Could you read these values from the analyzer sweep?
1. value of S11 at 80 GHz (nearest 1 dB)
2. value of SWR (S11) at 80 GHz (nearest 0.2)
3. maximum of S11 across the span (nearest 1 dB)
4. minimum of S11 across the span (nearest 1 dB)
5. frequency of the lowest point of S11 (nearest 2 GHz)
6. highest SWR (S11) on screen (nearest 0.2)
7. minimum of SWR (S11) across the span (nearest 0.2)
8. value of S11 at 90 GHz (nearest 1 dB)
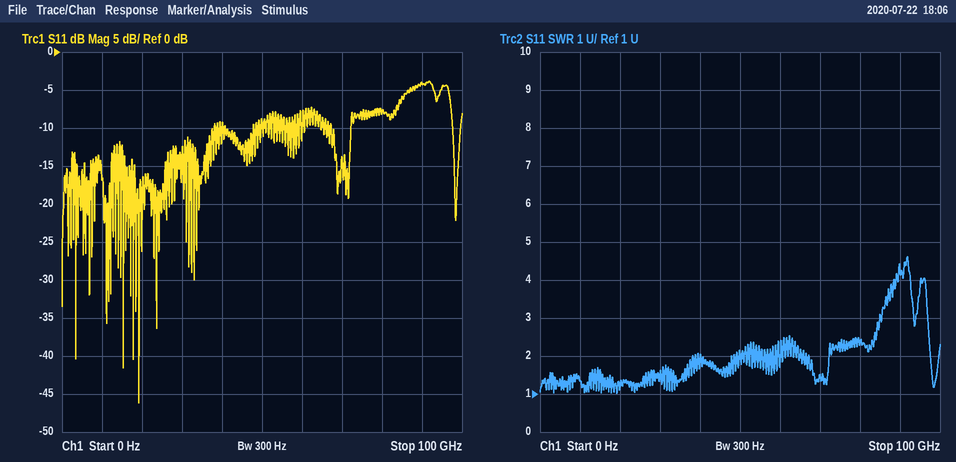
-8 dB
2.4
-4 dB
-46 dB
20 GHz
4.6
1.0
-4 dB
